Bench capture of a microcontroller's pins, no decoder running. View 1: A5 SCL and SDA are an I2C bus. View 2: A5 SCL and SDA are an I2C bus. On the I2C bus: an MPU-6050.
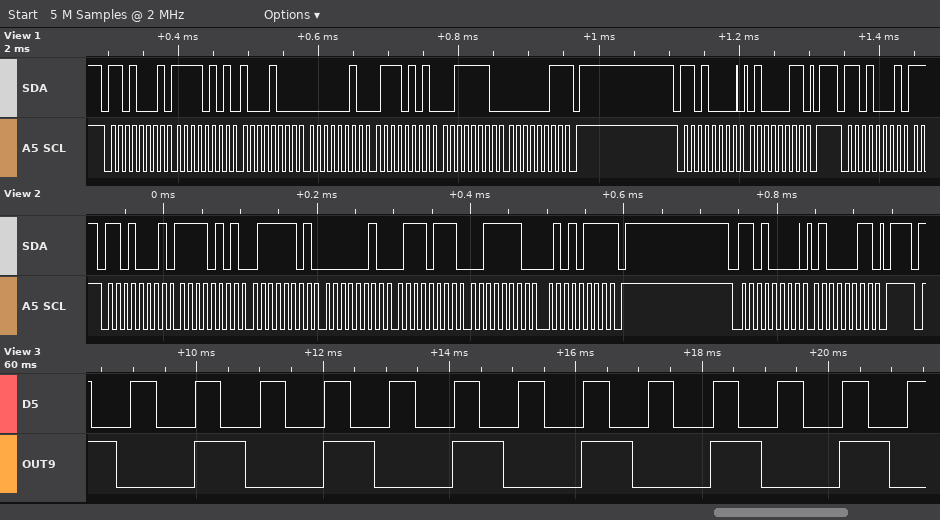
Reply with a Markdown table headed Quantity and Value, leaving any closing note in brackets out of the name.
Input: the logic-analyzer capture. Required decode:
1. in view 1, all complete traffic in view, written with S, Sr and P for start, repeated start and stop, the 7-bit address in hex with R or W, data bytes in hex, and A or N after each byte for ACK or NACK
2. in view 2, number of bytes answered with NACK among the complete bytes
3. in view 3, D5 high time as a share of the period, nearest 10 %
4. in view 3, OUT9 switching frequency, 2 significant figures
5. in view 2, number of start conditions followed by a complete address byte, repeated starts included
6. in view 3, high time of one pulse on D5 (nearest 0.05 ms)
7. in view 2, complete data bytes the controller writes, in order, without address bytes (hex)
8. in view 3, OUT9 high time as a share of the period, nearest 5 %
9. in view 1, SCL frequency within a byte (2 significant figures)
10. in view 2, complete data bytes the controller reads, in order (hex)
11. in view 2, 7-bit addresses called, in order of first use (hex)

| Quantity | Value |
|---|---|
| in view 1, all complete traffic in view, written with S, Sr and P for start, repeated start and stop, the 7-bit address in hex with R or W, data bytes in hex, and A or N after each byte for ACK or NACK | S 68R A F5 A 88 A 02 A 75 A 3E A 03 N P S 68W A 43 A P S 68R A |
| in view 2, number of bytes answered with NACK among the complete bytes | 1 |
| in view 3, D5 high time as a share of the period, nearest 10 % | 40 % |
| in view 3, OUT9 switching frequency, 2 significant figures | 490 Hz |
| in view 2, number of start conditions followed by a complete address byte, repeated starts included | 2 |
| in view 3, high time of one pulse on D5 | 0.40 ms |
| in view 2, complete data bytes the controller writes, in order, without address bytes | 43 |
| in view 3, OUT9 high time as a share of the period, nearest 5 % | 40 % |
| in view 1, SCL frequency within a byte | 100 kHz |
| in view 2, complete data bytes the controller reads, in order | F5 7D 02 77 3E 57 |
| in view 2, 7-bit addresses called, in order of first use | 0x68 |
